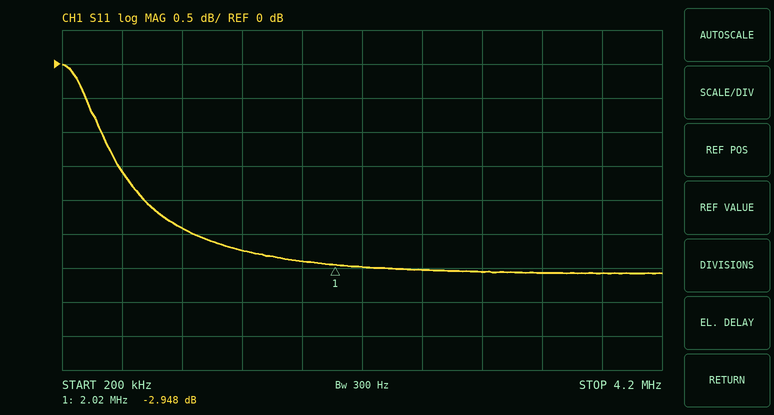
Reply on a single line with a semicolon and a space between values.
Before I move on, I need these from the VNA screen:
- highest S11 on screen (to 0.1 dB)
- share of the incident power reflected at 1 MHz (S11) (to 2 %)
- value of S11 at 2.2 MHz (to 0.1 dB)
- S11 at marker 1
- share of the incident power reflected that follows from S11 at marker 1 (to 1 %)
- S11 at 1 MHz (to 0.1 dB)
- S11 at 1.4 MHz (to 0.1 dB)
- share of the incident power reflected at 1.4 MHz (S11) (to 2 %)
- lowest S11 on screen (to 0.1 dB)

0.0 dB; 58 %; -3.0 dB; -2.948 dB; 51 %; -2.4 dB; -2.7 dB; 54 %; -3.1 dB
